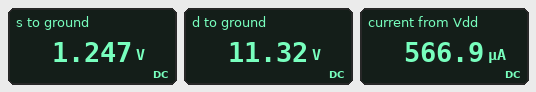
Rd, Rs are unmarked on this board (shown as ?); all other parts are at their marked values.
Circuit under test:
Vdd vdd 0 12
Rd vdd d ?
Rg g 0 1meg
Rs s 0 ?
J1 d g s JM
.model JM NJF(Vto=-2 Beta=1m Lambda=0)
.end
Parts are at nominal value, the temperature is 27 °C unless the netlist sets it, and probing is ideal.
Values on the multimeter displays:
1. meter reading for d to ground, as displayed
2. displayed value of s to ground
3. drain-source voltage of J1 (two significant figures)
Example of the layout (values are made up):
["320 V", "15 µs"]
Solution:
["11.32 V", "1.247 V", "10 V"]
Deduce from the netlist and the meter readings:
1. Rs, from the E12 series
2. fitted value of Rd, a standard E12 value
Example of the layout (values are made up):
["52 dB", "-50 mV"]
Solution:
["2.2 kΩ", "1.2 kΩ"]
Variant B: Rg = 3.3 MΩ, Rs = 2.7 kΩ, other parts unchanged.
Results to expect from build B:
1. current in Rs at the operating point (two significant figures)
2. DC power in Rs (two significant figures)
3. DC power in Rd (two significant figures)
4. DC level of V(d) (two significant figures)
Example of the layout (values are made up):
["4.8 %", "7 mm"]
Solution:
["480 µA", "630 µW", "280 µW", "11 V"]
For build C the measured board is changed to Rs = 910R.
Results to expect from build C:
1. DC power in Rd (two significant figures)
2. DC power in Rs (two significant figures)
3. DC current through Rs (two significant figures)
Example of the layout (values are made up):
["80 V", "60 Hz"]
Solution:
["1.4 mW", "1.0 mW", "1.1 mA"]
